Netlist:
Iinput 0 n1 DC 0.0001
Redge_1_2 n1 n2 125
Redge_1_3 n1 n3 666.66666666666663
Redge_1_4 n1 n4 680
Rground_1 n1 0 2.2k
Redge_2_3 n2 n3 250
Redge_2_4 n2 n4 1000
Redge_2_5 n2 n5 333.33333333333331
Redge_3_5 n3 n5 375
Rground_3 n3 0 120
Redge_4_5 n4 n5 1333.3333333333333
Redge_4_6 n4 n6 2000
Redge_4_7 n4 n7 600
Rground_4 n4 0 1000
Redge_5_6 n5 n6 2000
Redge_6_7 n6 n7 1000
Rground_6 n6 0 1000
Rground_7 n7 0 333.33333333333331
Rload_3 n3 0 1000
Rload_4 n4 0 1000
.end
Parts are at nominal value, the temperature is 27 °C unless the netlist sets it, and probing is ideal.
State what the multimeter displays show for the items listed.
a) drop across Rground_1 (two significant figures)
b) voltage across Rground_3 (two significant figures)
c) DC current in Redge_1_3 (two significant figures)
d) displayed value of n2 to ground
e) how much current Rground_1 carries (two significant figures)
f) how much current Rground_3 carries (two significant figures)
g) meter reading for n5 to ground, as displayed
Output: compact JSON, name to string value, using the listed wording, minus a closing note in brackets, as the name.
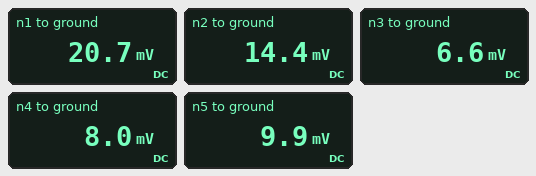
{"drop across Rground_1": "21 mV", "voltage across Rground_3": "6.6 mV", "DC current in Redge_1_3": "21 µA", "displayed value of n2 to ground": "14.4 mV", "how much current Rground_1 carries": "9.4 µA", "how much current Rground_3 carries": "55 µA", "meter reading for n5 to ground, as displayed": "9.9 mV"}
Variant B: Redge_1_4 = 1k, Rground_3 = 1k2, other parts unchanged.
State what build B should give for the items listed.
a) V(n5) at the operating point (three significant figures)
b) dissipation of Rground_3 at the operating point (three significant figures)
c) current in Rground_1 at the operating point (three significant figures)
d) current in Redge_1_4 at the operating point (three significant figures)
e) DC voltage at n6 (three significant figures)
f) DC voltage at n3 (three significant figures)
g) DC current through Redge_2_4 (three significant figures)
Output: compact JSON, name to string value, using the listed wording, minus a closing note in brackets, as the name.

{"V(n5) at the operating point": "21.3 mV", "dissipation of Rground_3 at the operating point": "365 nW", "current in Rground_1 at the operating point": "14.6 µA", "current in Redge_1_4 at the operating point": "19.7 µA", "DC voltage at n6": "7.27 mV", "DC voltage at n3": "20.9 mV", "DC current through Redge_2_4": "13.6 µA"}
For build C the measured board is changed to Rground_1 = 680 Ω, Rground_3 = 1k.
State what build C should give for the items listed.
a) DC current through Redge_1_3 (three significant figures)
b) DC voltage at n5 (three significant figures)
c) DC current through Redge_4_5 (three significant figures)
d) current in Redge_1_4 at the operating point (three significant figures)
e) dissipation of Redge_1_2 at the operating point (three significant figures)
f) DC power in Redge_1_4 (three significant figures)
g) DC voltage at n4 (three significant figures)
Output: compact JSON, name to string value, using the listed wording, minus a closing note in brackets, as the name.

{"DC current through Redge_1_3": "12.4 µA", "DC voltage at n5": "15.2 mV", "DC current through Redge_4_5": "4.00 µA", "current in Redge_1_4 at the operating point": "19.2 µA", "dissipation of Redge_1_2 at the operating point": "150 nW", "DC power in Redge_1_4": "251 nW", "DC voltage at n4": "9.88 mV"}
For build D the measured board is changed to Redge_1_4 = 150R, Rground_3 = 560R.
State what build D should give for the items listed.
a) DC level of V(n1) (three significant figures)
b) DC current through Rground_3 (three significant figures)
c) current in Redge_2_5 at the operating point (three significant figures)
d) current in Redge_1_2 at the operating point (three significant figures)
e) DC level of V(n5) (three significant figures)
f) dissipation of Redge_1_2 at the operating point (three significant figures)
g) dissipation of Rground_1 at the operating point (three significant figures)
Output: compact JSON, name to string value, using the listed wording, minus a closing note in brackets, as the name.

{"DC level of V(n1)": "21.8 mV", "DC current through Rground_3": "23.5 µA", "current in Redge_2_5 at the operating point": "8.90 µA", "current in Redge_1_2 at the operating point": "31.0 µA", "DC level of V(n5)": "15.0 mV", "dissipation of Redge_1_2 at the operating point": "120 nW", "dissipation of Rground_1 at the operating point": "216 nW"}
